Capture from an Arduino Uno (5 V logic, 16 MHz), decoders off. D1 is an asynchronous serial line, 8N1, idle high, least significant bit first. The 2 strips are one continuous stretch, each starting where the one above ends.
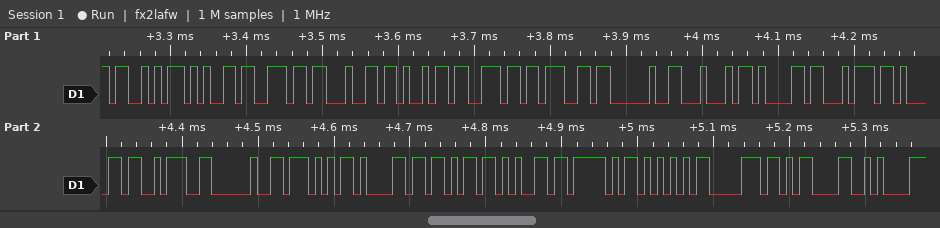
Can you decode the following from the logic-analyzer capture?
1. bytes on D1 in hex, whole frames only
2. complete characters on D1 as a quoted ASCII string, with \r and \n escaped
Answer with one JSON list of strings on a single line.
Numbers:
["0x53 0x65 0x6E 0x64 0x69 0x6E 0x67 0x20 0x44 0x61 0x74 0x61 0x3A 0x20 0x57 0x61 0x6B 0x65 0x5F 0x55 0x70 0x0D 0x0A", "\"Sending Data: Wake_Up\\r\\n\""]
